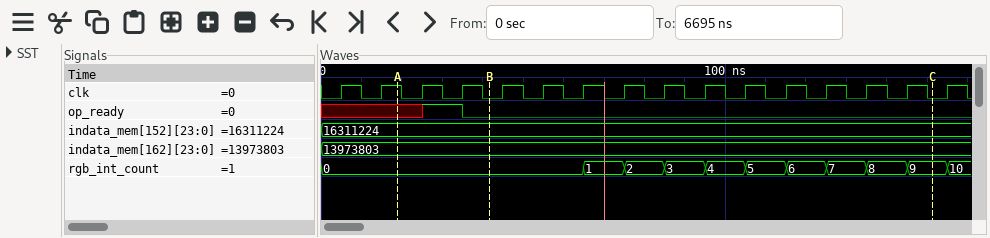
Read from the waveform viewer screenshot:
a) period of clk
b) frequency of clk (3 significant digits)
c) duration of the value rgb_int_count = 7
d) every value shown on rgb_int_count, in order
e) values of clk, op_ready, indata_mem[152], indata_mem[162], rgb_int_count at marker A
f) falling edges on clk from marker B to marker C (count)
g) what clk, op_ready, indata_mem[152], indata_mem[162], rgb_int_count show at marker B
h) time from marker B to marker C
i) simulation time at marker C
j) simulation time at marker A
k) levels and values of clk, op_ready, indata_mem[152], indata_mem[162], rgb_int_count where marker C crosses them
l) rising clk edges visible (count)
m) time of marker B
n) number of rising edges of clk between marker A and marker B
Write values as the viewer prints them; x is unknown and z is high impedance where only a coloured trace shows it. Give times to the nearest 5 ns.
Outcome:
10 ns
100 MHz
10 ns
0, 1, 2, 3, 4, 5, 6, 7, 8, 9, 10
clk=1, op_ready=x, indata_mem[152]=16311224, indata_mem[162]=13973803, rgb_int_count=0
11
clk=0, op_ready=0, indata_mem[152]=16311224, indata_mem[162]=13973803, rgb_int_count=0
110 ns
150 ns
20 ns
clk=0, op_ready=0, indata_mem[152]=16311224, indata_mem[162]=13973803, rgb_int_count=9
16
40 ns
2
